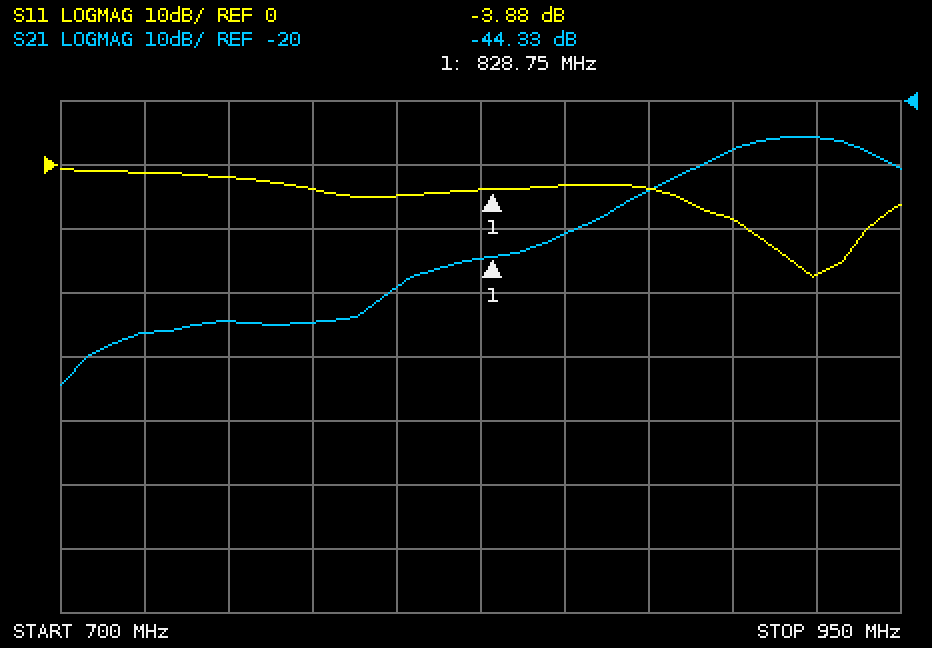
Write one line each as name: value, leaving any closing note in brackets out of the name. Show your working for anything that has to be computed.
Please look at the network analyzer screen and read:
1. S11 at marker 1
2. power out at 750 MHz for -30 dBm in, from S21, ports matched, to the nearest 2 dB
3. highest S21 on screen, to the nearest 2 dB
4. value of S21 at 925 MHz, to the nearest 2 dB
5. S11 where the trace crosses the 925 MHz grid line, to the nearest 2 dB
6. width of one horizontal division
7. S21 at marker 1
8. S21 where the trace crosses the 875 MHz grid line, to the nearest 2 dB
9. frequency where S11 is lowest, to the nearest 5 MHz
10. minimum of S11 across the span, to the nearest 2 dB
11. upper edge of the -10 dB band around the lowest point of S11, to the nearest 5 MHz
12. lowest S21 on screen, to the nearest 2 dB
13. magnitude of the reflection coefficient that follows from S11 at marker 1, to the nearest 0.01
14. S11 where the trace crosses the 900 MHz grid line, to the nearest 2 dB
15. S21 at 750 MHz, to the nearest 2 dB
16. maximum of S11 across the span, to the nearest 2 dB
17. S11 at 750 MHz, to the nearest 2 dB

S11 at marker 1: -3.88 dB
power out at 750 MHz for -30 dBm in, from S21, ports matched, to the nearest 2 dB: -30 dBm + (-54 dB) = -84 dBm
highest S21 on screen, to the nearest 2 dB: -26 dB
value of S21 at 925 MHz, to the nearest 2 dB: -26 dB
S11 where the trace crosses the 925 MHz grid line, to the nearest 2 dB: -18 dB
width of one horizontal division: 25 MHz
S21 at marker 1: -44.33 dB
S21 where the trace crosses the 875 MHz grid line, to the nearest 2 dB: -34 dB
frequency where S11 is lowest, to the nearest 5 MHz: 925 MHz
minimum of S11 across the span, to the nearest 2 dB: -18 dB
upper edge of the -10 dB band around the lowest point of S11, to the nearest 5 MHz: 940 MHz
lowest S21 on screen, to the nearest 2 dB: -64 dB
magnitude of the reflection coefficient that follows from S11 at marker 1, to the nearest 0.01: 10^(-3.88/20) ≈ 0.64
S11 where the trace crosses the 900 MHz grid line, to the nearest 2 dB: -8 dB
S21 at 750 MHz, to the nearest 2 dB: -54 dB
maximum of S11 across the span, to the nearest 2 dB: 0 dB
S11 at 750 MHz, to the nearest 2 dB: -2 dB
